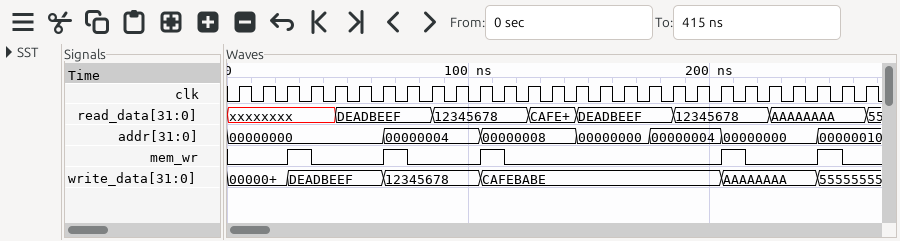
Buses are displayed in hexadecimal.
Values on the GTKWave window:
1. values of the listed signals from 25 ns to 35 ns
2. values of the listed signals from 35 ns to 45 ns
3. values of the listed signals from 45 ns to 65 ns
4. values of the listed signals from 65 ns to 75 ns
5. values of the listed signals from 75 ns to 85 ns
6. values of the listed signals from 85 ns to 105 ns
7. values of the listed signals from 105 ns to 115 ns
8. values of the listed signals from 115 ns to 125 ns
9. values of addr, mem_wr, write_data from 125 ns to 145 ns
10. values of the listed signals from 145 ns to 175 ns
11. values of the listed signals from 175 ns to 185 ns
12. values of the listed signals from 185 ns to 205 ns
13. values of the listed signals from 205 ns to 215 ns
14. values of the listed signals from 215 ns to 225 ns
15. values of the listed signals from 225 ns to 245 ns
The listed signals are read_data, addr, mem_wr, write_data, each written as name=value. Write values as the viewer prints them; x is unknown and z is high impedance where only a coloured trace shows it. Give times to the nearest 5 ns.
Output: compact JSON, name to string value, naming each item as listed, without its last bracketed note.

{"values of the listed signals from 25 ns to 35 ns": "read_data=xxxxxxxx, addr=00000000, mem_wr=1, write_data=DEADBEEF", "values of the listed signals from 35 ns to 45 ns": "read_data=xxxxxxxx, addr=00000000, mem_wr=0, write_data=DEADBEEF", "values of the listed signals from 45 ns to 65 ns": "read_data=DEADBEEF, addr=00000000, mem_wr=0, write_data=DEADBEEF", "values of the listed signals from 65 ns to 75 ns": "read_data=DEADBEEF, addr=00000004, mem_wr=1, write_data=12345678", "values of the listed signals from 75 ns to 85 ns": "read_data=DEADBEEF, addr=00000004, mem_wr=0, write_data=12345678", "values of the listed signals from 85 ns to 105 ns": "read_data=12345678, addr=00000004, mem_wr=0, write_data=12345678", "values of the listed signals from 105 ns to 115 ns": "read_data=12345678, addr=00000008, mem_wr=1, write_data=CAFEBABE", "values of the listed signals from 115 ns to 125 ns": "read_data=12345678, addr=00000008, mem_wr=0, write_data=CAFEBABE", "values of addr, mem_wr, write_data from 125 ns to 145 ns": "addr=00000008, mem_wr=0, write_data=CAFEBABE", "values of the listed signals from 145 ns to 175 ns": "read_data=DEADBEEF, addr=00000000, mem_wr=0, write_data=CAFEBABE", "values of the listed signals from 175 ns to 185 ns": "read_data=DEADBEEF, addr=00000004, mem_wr=0, write_data=CAFEBABE", "values of the listed signals from 185 ns to 205 ns": "read_data=12345678, addr=00000004, mem_wr=0, write_data=CAFEBABE", "values of the listed signals from 205 ns to 215 ns": "read_data=12345678, addr=00000000, mem_wr=1, write_data=AAAAAAAA", "values of the listed signals from 215 ns to 225 ns": "read_data=12345678, addr=00000000, mem_wr=0, write_data=AAAAAAAA", "values of the listed signals from 225 ns to 245 ns": "read_data=AAAAAAAA, addr=00000000, mem_wr=0, write_data=AAAAAAAA"}
